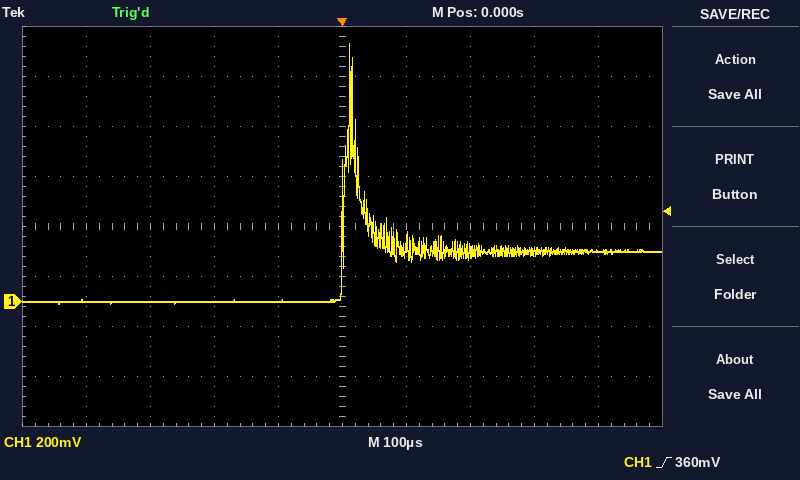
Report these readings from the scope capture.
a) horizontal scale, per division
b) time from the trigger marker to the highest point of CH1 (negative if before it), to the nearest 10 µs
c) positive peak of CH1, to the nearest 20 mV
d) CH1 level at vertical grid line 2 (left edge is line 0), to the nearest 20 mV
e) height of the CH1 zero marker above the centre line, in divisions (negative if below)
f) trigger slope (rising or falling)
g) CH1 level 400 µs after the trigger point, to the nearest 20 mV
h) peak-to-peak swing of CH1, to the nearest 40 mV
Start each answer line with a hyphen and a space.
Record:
- 100 µs
- +10 µs
- 1.04 V
- 0 mV
- -1.5 div
- rising
- 200 mV
- 1.04 V
